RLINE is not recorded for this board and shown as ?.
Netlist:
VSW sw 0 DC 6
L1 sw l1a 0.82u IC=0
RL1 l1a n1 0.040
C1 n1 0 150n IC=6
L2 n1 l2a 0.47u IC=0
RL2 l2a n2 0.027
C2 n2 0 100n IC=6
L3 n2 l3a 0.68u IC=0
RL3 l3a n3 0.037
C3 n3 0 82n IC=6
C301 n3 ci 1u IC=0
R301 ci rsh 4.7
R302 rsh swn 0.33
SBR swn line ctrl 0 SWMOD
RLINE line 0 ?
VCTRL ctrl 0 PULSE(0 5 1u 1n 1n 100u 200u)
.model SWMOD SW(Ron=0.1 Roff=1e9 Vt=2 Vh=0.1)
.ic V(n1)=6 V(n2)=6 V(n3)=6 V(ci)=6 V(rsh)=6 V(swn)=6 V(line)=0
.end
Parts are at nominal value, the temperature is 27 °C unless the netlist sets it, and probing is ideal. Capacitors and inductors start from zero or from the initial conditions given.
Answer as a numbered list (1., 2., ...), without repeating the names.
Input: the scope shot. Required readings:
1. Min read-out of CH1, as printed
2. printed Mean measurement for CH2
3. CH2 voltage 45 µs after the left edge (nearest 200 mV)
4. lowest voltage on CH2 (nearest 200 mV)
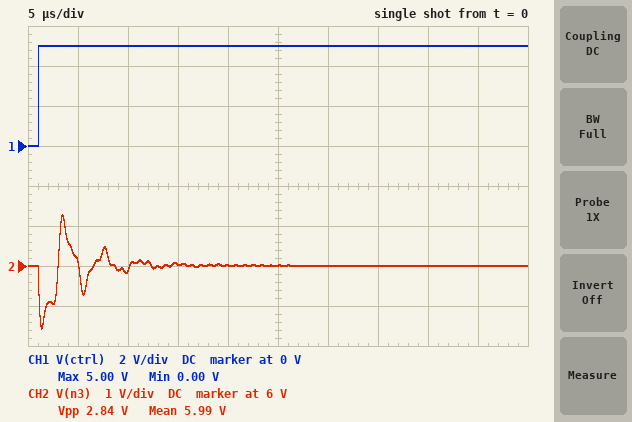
1. 0.00 V
2. 5.99 V
3. 6.0 V
4. 4.4 V
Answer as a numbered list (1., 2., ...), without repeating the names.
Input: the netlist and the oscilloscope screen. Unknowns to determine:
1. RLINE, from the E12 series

1. 3.9 Ω
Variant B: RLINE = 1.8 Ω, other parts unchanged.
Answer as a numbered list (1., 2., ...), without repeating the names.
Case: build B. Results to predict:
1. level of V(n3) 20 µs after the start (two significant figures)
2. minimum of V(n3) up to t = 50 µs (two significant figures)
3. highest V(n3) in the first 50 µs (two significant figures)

1. 6.0 V
2. 4.1 V
3. 7.4 V
